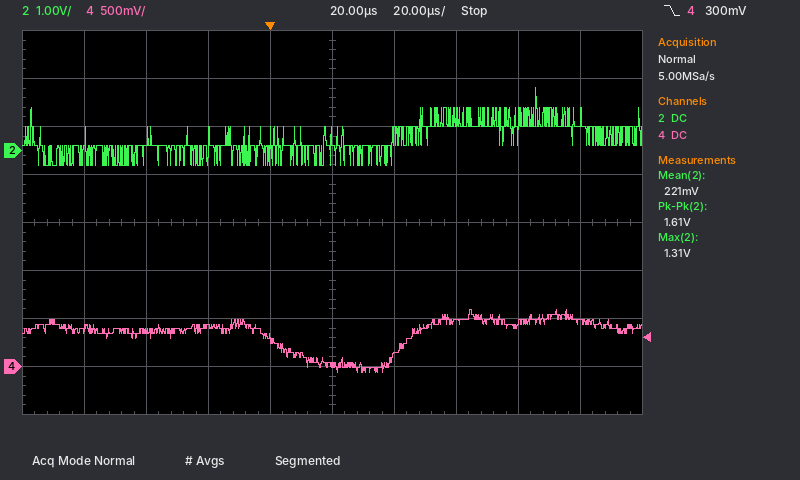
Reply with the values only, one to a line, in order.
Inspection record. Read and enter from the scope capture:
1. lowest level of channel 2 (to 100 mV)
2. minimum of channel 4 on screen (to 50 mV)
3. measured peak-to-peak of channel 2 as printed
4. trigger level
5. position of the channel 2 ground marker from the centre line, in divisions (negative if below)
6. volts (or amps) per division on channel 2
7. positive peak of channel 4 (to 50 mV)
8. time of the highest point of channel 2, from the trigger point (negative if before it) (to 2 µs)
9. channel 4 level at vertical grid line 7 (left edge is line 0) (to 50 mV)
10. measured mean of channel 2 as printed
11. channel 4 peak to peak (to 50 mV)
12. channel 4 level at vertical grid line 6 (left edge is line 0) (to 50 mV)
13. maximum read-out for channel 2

-300 mV
-50 mV
1.61 V
300 mV
+1.5 div
1 V
600 mV
+86 µs
500 mV
221 mV
650 mV
100 mV
1.31 V
